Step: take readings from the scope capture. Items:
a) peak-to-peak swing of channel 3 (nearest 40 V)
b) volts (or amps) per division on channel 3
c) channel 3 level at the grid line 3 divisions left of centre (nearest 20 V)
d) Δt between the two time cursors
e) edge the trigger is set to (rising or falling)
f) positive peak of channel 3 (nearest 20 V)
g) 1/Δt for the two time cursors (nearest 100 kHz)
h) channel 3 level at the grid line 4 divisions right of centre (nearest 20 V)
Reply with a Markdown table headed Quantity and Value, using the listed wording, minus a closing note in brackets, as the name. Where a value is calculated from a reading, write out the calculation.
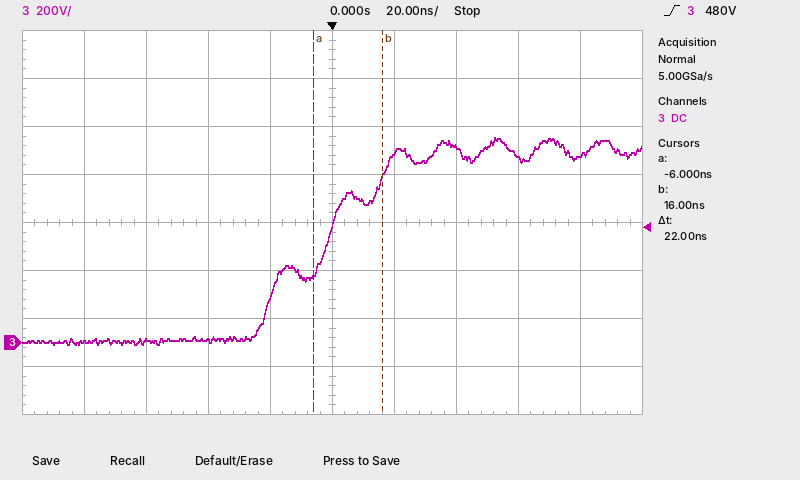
| Quantity | Value |
|---|---|
| peak-to-peak swing of channel 3 | 880 V |
| volts (or amps) per division on channel 3 | 200 V |
| channel 3 level at the grid line 3 divisions left of centre | 0 V |
| Δt between the two time cursors | 22 ns |
| edge the trigger is set to | rising |
| positive peak of channel 3 | 860 V |
| 1/Δt for the two time cursors | 1 / 22 ns ≈ 45.5 MHz |
| channel 3 level at the grid line 4 divisions right of centre | 780 V |
